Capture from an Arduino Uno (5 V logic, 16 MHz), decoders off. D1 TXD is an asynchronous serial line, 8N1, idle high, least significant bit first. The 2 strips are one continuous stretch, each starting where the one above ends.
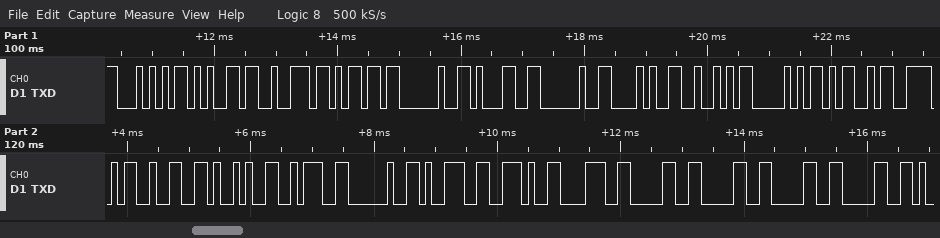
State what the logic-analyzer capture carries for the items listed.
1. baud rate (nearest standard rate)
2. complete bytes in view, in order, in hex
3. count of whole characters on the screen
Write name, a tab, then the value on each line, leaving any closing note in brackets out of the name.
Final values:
baud rate	9600 baud
complete bytes in view, in order, in hex	0x54 0x65 0x72 0x6D 0x20 0x31 0x20 0x28 0x52 0x50 0x4D 0x5E 0x32 0x29 0x3A 0x20 0x39 0x2E 0x38 0x30 0x30 0x30 0x30
count of whole characters on the screen	23
